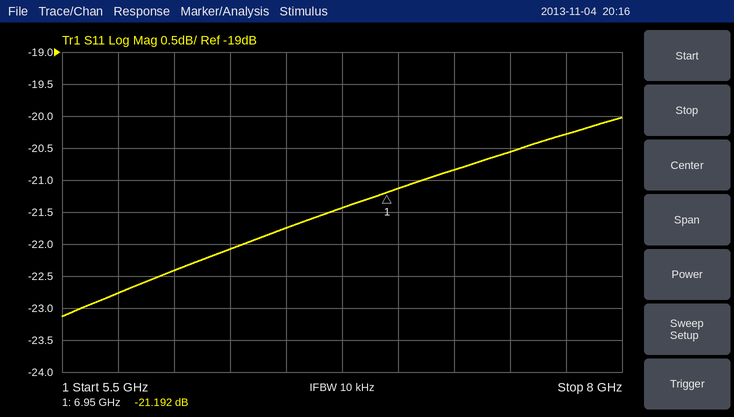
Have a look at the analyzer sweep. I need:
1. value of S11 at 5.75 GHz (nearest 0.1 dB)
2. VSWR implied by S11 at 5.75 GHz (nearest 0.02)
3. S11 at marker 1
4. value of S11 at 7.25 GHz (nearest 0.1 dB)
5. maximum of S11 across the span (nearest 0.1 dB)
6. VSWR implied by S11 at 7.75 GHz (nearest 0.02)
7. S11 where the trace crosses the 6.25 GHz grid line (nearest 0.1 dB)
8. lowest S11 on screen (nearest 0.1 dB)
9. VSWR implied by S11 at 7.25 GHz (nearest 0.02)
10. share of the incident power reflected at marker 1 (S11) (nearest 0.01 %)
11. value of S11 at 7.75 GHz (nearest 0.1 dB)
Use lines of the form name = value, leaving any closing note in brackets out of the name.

value of S11 at 5.75 GHz = -22.8 dB
VSWR implied by S11 at 5.75 GHz = 1.16
S11 at marker 1 = -21.192 dB
value of S11 at 7.25 GHz = -20.8 dB
maximum of S11 across the span = -20.0 dB
VSWR implied by S11 at 7.75 GHz = 1.22
S11 where the trace crosses the 6.25 GHz grid line = -22.1 dB
lowest S11 on screen = -23.1 dB
VSWR implied by S11 at 7.25 GHz = 1.20
share of the incident power reflected at marker 1 (S11) = 0.76 %
value of S11 at 7.75 GHz = -20.3 dB
